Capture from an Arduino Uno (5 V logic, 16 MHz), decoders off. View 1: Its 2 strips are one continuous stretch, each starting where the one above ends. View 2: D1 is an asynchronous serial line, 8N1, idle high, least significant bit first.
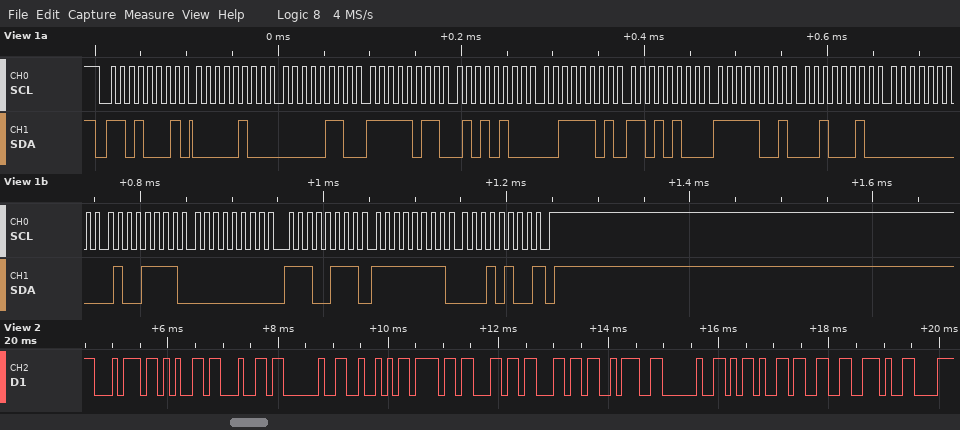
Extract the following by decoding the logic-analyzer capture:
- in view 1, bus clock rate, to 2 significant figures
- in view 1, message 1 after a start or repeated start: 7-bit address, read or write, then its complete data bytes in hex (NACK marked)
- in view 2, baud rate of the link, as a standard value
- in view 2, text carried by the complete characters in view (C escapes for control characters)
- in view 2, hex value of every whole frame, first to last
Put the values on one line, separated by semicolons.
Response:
100 kHz; 0x68 read: 04 06 FB 54 3D D4 F9 22 00 4F 00 E7 FF 14 NACK; 9600 baud; "ted Roll: -3."; 74 65 64 20 52 6F 6C 6C 3A 20 2D 33 2E
